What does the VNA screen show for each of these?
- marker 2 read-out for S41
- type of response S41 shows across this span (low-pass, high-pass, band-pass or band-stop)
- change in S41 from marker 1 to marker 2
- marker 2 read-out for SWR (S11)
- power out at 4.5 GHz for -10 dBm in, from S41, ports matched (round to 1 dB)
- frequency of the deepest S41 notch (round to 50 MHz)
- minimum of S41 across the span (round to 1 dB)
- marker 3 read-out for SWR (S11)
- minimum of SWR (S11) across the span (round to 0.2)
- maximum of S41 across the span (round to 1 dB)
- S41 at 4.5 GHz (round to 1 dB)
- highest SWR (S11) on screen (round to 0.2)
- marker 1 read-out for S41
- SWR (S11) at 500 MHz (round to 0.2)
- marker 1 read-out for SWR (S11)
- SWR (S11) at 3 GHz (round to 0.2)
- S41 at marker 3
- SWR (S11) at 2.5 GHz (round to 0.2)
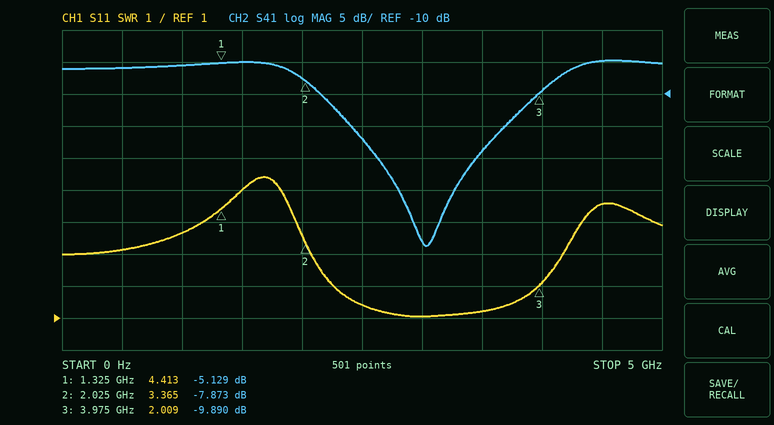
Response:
-7.873 dB
band-stop
-2.744 dB
3.365
-15 dBm
3.05 GHz
-34 dB
2.009
1.0
-5 dB
-5 dB
5.4
-5.129 dB
3.2
4.413
1.0
-9.890 dB
1.4
